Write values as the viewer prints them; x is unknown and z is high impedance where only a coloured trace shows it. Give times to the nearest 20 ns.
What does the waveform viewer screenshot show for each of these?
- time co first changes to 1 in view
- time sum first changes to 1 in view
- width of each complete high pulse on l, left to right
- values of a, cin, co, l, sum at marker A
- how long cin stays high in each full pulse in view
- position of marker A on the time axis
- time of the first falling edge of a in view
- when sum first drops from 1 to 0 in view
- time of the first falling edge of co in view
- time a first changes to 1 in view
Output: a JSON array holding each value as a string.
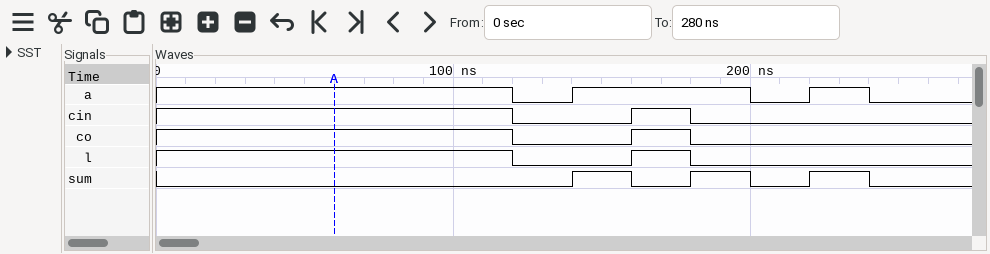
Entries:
["160 ns", "140 ns", "20 ns", "a=1, cin=1, co=1, l=1, sum=0", "20 ns", "60 ns", "120 ns", "160 ns", "120 ns", "140 ns"]
